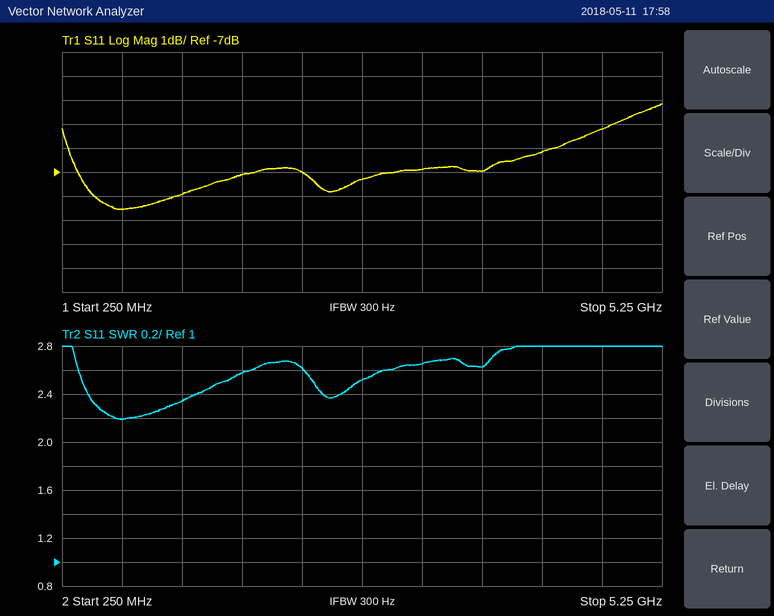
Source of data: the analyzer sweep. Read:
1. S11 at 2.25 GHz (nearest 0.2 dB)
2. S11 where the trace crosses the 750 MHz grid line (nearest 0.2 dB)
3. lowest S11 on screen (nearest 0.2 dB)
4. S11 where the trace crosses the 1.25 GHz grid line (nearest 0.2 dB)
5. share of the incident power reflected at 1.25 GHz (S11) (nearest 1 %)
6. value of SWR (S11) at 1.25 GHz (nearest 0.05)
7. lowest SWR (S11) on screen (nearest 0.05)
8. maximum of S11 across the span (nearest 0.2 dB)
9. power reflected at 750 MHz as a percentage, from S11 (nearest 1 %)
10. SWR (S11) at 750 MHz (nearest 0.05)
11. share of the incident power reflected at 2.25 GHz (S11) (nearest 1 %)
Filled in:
-7.0 dB
-8.6 dB
-8.6 dB
-8.0 dB
16 %
2.35
2.20
-4.2 dB
14 %
2.20
20 %
